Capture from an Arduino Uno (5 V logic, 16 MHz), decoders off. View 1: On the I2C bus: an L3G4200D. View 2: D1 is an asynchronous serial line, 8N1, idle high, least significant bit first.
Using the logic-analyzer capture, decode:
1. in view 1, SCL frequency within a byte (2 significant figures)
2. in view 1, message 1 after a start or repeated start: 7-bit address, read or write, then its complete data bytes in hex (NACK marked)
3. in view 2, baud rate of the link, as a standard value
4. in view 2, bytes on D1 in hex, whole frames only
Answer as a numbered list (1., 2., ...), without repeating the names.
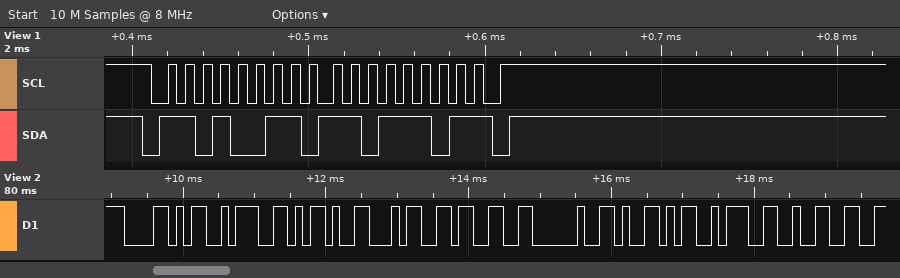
1. 100 kHz
2. 0x69 read: DD NACK
3. 9600 baud
4. 0x58 0x3A 0x2D 0x34 0x33 0x20 0x59 0x3A 0x32
